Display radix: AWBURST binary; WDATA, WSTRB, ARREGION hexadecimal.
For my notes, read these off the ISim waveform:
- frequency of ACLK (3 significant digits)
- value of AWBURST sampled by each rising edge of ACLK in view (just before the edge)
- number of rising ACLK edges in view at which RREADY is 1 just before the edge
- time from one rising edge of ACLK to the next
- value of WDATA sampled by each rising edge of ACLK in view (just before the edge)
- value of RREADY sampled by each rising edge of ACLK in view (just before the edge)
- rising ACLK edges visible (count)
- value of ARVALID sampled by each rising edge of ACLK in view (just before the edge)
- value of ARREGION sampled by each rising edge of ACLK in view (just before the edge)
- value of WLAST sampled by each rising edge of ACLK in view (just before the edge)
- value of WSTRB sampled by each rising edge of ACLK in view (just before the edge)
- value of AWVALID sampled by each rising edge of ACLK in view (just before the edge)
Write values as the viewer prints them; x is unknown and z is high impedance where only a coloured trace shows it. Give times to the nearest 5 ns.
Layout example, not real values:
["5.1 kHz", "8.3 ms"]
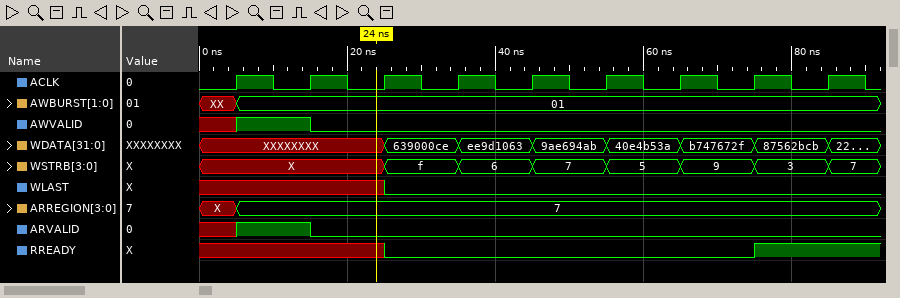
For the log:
["100 MHz", "XX, 01, 01, 01, 01, 01, 01, 01, 01", "1", "10 ns", "XXXXXXXX, XXXXXXXX, XXXXXXXX, 639000ce, ee9d1063, 9ae694ab, 40e4b53a, b747672f, 87562bcb", "x x x 0 0 0 0 0 1", "9", "x 1 0 0 0 0 0 0 0", "X, 7, 7, 7, 7, 7, 7, 7, 7", "x x x 0 0 0 0 0 0", "X, X, X, f, 6, 7, 5, 9, 3", "x 1 0 0 0 0 0 0 0"]
